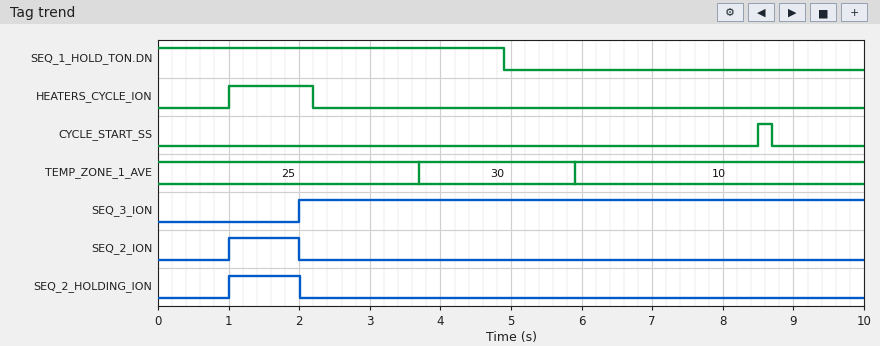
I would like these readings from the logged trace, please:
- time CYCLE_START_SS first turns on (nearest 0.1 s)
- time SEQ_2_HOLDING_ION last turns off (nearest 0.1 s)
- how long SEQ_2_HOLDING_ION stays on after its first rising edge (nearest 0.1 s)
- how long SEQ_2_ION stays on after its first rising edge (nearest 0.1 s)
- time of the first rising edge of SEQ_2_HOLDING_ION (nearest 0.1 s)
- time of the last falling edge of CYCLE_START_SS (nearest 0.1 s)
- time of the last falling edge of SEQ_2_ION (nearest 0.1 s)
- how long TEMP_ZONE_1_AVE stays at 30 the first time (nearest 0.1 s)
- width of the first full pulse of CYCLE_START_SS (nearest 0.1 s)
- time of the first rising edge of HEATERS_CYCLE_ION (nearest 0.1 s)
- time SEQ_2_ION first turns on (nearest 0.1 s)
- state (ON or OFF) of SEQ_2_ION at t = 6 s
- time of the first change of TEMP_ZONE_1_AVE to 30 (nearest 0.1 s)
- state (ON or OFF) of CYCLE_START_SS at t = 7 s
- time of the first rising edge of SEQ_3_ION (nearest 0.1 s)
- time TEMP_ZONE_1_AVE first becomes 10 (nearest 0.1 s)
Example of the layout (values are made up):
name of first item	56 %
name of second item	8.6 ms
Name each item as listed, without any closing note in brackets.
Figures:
time CYCLE_START_SS first turns on	8.5 s
time SEQ_2_HOLDING_ION last turns off	2.0 s
how long SEQ_2_HOLDING_ION stays on after its first rising edge	1.0 s
how long SEQ_2_ION stays on after its first rising edge	1.0 s
time of the first rising edge of SEQ_2_HOLDING_ION	1.0 s
time of the last falling edge of CYCLE_START_SS	8.7 s
time of the last falling edge of SEQ_2_ION	2.0 s
how long TEMP_ZONE_1_AVE stays at 30 the first time	2.2 s
width of the first full pulse of CYCLE_START_SS	0.2 s
time of the first rising edge of HEATERS_CYCLE_ION	1.0 s
time SEQ_2_ION first turns on	1.0 s
state (ON or OFF) of SEQ_2_ION at t = 6 s	OFF
time of the first change of TEMP_ZONE_1_AVE to 30	3.7 s
state (ON or OFF) of CYCLE_START_SS at t = 7 s	OFF
time of the first rising edge of SEQ_3_ION	2.0 s
time TEMP_ZONE_1_AVE first becomes 10	5.9 s
